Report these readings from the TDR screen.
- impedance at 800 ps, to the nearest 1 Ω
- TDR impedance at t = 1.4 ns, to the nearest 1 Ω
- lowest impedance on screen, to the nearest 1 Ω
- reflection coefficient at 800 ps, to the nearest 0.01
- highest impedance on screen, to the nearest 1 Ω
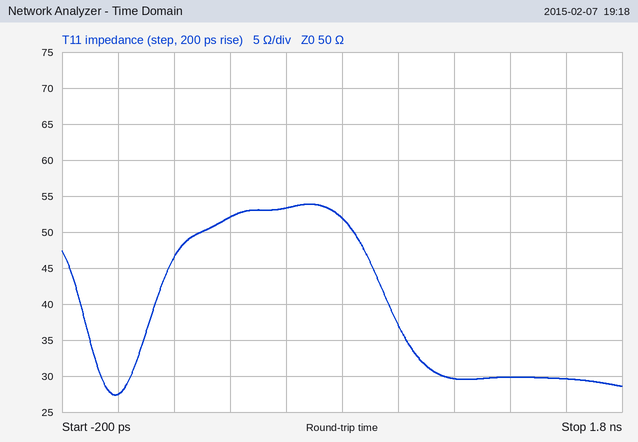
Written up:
52 Ω
30 Ω
27 Ω
+0.02
54 Ω
